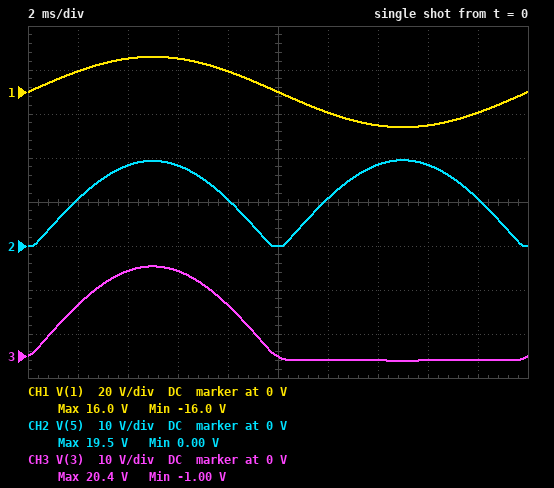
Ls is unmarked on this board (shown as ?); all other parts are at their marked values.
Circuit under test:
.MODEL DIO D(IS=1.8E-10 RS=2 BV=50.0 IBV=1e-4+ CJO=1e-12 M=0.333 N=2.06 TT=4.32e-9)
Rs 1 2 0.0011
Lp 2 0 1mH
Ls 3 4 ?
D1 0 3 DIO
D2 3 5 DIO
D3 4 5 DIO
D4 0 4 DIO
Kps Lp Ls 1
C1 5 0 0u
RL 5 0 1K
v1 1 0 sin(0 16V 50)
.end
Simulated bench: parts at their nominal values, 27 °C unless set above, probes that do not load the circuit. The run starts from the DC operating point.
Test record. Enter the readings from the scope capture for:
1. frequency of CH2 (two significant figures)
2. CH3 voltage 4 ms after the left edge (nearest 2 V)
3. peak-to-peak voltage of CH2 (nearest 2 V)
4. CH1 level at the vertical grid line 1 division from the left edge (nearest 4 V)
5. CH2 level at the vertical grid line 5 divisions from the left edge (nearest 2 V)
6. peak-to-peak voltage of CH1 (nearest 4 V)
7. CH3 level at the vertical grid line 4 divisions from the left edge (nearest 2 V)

100 Hz
20 V
20 V
8 V
0 V
32 V
12 V
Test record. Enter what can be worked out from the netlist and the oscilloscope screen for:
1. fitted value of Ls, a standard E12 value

1.8 mH
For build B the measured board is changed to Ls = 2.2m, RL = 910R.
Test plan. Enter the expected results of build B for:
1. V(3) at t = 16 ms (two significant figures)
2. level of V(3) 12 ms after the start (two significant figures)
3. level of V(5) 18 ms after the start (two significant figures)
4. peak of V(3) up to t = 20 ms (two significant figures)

-1.0 V
-990 mV
12 V
23 V
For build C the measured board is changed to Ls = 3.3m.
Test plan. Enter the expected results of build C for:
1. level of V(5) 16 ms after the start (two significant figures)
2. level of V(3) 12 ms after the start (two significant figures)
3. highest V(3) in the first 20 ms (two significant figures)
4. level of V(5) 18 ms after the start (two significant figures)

26 V
-1.0 V
28 V
15 V
